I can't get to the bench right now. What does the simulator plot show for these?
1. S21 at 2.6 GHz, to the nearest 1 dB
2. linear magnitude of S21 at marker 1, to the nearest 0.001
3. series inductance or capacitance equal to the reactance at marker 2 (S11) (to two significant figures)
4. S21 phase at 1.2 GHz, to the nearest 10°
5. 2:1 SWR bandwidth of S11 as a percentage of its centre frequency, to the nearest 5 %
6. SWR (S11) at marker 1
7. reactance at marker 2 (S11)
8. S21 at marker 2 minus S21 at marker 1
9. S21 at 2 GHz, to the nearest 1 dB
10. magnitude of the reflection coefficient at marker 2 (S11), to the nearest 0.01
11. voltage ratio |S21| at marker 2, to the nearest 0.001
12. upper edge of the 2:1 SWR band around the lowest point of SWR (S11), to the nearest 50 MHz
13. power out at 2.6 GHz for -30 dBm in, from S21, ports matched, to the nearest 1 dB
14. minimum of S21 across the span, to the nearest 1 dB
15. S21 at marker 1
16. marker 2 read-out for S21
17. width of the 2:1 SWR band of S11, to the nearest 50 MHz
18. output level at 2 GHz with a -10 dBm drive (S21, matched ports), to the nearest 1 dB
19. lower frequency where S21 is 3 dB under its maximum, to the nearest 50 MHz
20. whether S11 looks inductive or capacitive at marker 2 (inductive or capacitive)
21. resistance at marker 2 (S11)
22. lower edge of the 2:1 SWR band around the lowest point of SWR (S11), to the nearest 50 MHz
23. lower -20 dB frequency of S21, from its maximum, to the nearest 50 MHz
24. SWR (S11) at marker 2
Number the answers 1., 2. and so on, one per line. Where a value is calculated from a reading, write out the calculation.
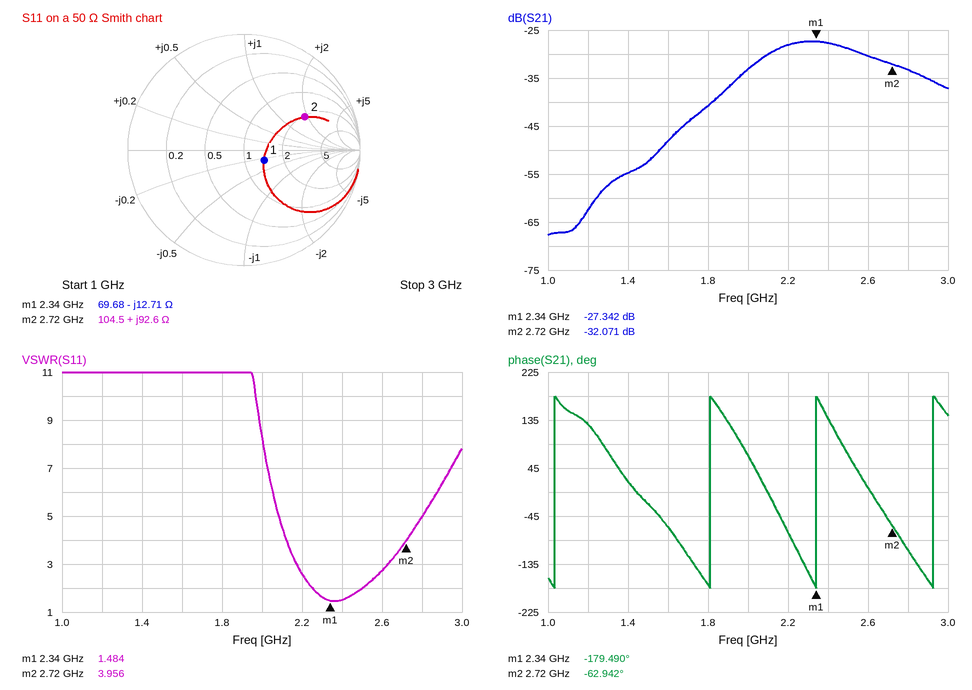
1. -30 dB
2. 10^(-27.342/20) ≈ 0.043
3. L = 92.6 Ω/(2π × 2.72 GHz) ≈ 5.4 nH
4. 130°
5. 250 MHz / 2.375 GHz ≈ 10 %
6. 1.484
7. +92.6 Ω
8. -32.071 − (-27.342) = -4.729 dB
9. -33 dB
10. 0.60
11. 10^(-32.071/20) ≈ 0.025
12. 2.50 GHz
13. -30 dBm + (-30 dB) = -60 dBm
14. -68 dB
15. -27.342 dB
16. -32.071 dB
17. 2.50 GHz − 2.25 GHz = 250 MHz
18. -10 dBm + (-33 dB) = -43 dBm
19. 2.10 GHz
20. inductive
21. 104.5 Ω
22. 2.25 GHz
23. 1.60 GHz
24. 3.956
